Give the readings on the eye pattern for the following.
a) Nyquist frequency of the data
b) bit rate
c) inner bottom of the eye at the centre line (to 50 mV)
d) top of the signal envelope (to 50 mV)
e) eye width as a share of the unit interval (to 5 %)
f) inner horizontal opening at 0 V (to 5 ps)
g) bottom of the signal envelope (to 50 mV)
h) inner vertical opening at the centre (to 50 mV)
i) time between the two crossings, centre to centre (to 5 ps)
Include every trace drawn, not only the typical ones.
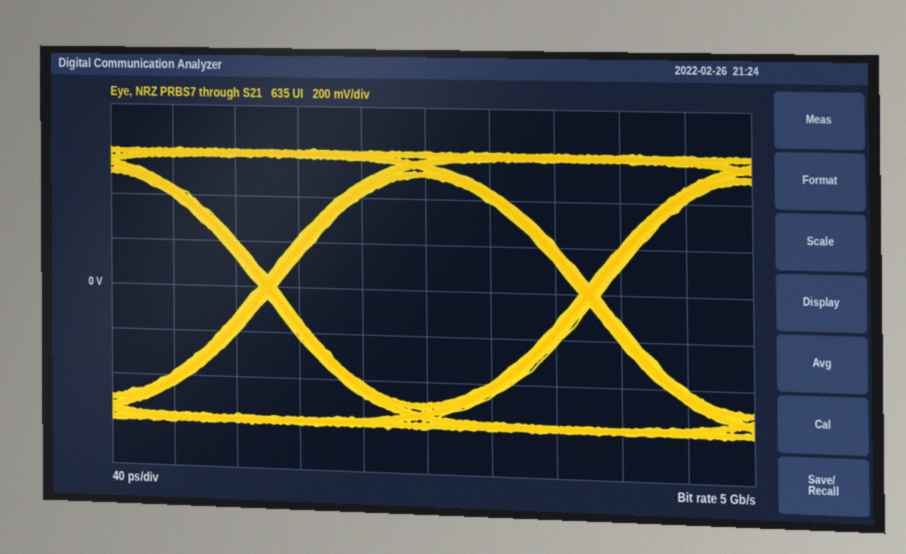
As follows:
2.5 GHz
5 Gb/s
-500 mV
600 mV
95 %
190 ps
-600 mV
1.00 V
200 ps
